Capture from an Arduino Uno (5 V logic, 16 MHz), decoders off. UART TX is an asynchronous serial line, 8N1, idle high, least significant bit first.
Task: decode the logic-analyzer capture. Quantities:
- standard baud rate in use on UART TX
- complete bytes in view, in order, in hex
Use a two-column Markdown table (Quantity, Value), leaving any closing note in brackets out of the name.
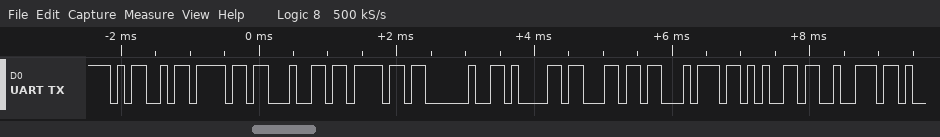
| Quantity | Value |
|---|---|
| standard baud rate in use on UART TX | 9600 baud |
| complete bytes in view, in order, in hex | 0x4D 0x6F 0x64 0x6F 0x20 0x61 0x6C 0x74 0x65 0x72 |
